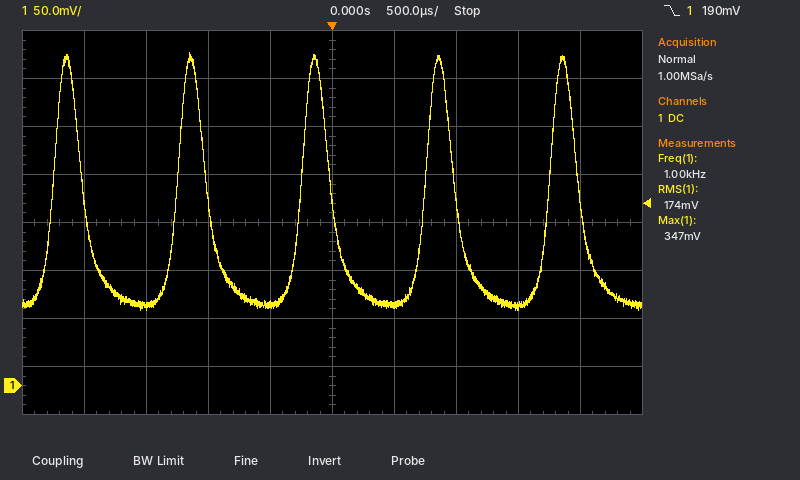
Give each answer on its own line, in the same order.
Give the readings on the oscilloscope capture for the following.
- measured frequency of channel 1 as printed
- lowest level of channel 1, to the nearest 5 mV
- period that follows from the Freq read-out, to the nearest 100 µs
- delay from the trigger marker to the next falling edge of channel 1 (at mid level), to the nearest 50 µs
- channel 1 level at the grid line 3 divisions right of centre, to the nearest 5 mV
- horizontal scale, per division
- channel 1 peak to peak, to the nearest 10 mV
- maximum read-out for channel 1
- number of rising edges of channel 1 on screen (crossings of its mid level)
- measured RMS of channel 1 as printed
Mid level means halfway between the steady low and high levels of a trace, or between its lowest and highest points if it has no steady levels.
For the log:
1.00 kHz
80 mV
1.0 ms
1.00 ms
85 mV
500 µs
270 mV
347 mV
5
174 mV
